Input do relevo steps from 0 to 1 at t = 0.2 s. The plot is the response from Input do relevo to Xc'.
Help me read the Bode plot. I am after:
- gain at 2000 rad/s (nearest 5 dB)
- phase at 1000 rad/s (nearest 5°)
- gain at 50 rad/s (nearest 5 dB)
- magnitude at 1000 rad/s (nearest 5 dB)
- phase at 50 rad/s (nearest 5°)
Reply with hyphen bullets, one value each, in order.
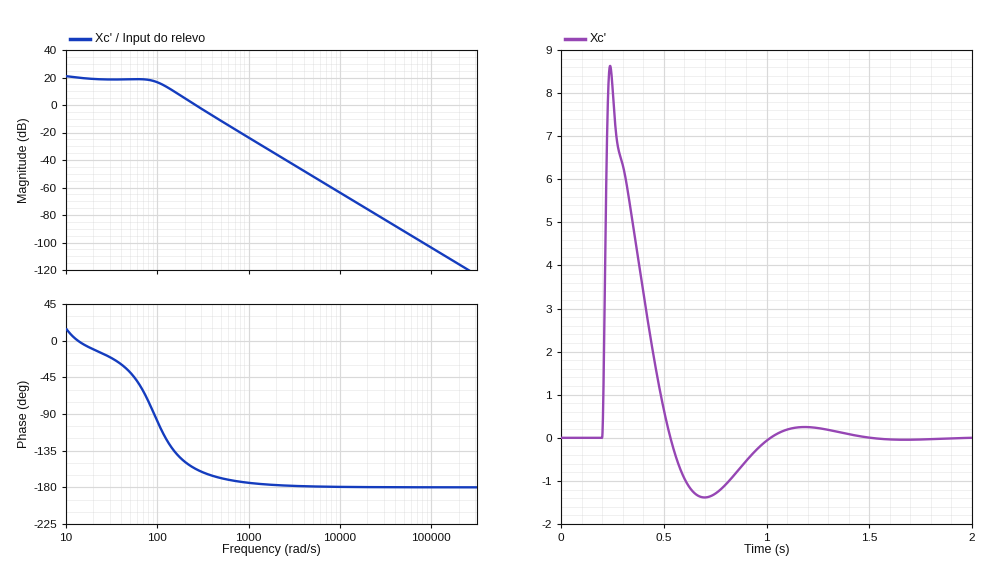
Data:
- -35 dB
- -175°
- 20 dB
- -25 dB
- -40°
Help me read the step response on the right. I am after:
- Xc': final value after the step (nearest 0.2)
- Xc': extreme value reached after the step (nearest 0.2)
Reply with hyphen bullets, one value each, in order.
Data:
- 0.0
- 8.6
